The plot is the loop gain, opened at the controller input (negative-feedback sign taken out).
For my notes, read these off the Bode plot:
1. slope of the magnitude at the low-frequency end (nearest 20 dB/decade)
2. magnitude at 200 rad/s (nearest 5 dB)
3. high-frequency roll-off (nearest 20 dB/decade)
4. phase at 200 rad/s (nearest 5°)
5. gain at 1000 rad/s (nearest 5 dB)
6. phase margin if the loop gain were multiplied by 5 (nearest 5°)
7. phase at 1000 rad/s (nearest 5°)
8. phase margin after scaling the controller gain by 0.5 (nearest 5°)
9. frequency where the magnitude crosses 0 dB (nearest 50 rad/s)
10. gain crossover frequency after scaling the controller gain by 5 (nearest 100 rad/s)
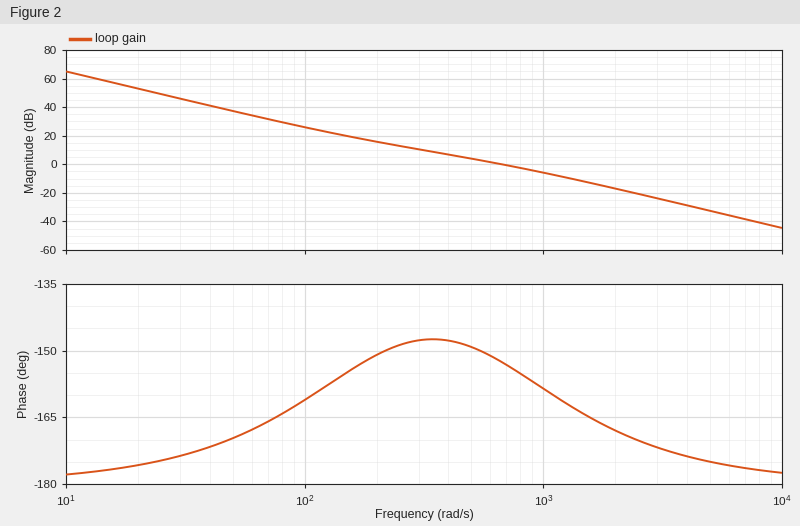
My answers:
-40 dB/decade
15 dB
-40 dB/decade
-150°
-5 dB
15°
-160°
30°
650 rad/s
1700 rad/s
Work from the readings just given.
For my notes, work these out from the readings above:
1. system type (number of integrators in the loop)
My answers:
2
